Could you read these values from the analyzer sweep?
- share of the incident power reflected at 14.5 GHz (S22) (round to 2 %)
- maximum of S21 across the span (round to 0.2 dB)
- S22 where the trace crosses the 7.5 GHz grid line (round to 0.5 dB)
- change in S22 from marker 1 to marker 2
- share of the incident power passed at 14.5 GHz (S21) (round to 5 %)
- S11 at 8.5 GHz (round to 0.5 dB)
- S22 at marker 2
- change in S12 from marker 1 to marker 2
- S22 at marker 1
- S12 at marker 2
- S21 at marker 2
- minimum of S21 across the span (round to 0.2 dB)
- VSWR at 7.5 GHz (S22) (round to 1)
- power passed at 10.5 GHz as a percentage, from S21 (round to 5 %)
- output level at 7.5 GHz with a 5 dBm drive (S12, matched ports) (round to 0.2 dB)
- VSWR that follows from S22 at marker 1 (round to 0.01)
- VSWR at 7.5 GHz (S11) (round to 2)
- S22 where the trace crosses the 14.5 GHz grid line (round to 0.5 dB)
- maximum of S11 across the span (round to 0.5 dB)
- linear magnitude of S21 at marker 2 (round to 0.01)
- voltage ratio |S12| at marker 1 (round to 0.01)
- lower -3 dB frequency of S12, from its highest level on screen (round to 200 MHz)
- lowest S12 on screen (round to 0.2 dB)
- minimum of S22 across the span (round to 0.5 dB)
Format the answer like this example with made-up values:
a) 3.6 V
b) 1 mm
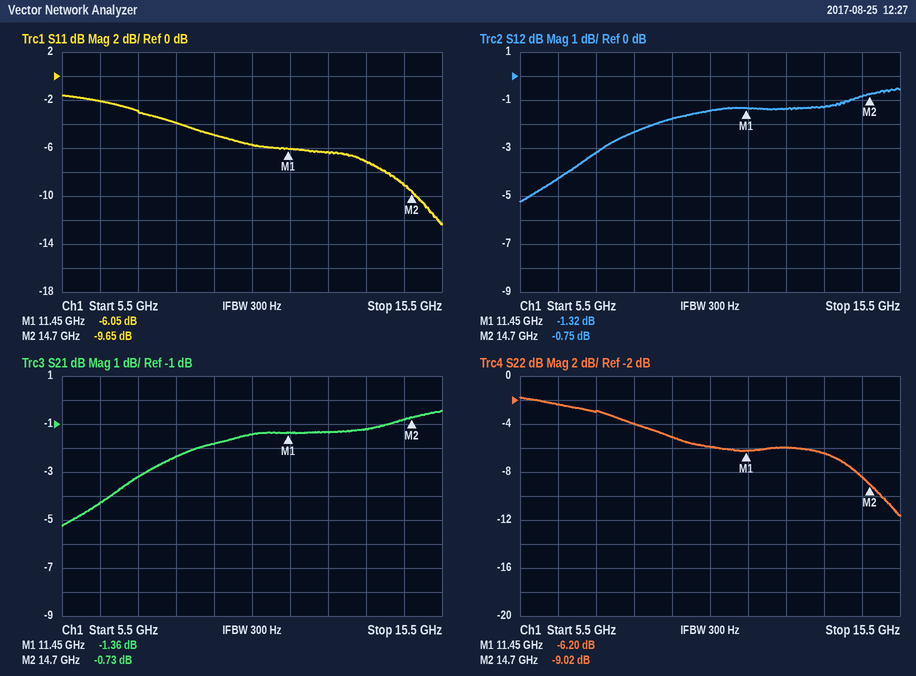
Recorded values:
a) 14 %
b) -0.4 dB
c) -3.0 dB
d) -2.82 dB
e) 85 %
f) -4.0 dB
g) -9.02 dB
h) 0.57 dB
i) -6.20 dB
j) -0.75 dB
k) -0.73 dB
l) -5.2 dB
m) 6
n) 70 %
o) 1.8 dBm
p) 2.92
q) 6
r) -8.5 dB
s) -1.5 dB
t) 0.92
u) 0.86
v) 7.2 GHz
w) -5.2 dB
x) -11.5 dB
